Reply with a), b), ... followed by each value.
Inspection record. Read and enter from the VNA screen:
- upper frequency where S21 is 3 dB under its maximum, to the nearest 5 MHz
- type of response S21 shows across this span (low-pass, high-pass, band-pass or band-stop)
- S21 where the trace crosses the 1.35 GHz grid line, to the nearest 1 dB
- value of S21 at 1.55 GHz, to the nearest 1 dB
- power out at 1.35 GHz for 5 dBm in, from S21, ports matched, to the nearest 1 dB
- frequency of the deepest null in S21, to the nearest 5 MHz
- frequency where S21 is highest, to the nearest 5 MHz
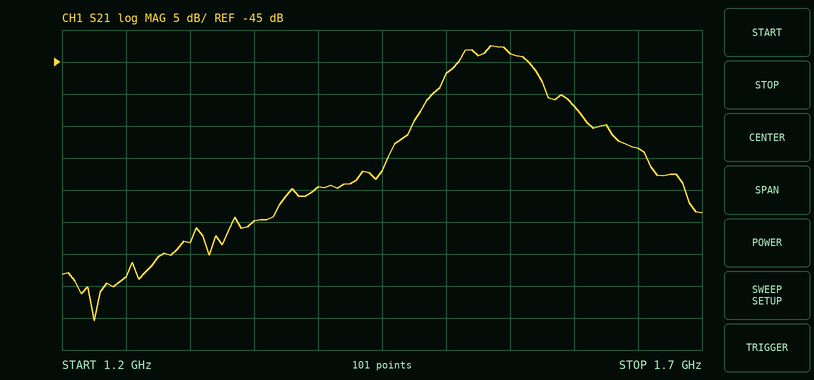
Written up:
a) 1.565 GHz
b) band-pass
c) -70 dB
d) -44 dB
e) -65 dBm
f) 1.225 GHz
g) 1.535 GHz
